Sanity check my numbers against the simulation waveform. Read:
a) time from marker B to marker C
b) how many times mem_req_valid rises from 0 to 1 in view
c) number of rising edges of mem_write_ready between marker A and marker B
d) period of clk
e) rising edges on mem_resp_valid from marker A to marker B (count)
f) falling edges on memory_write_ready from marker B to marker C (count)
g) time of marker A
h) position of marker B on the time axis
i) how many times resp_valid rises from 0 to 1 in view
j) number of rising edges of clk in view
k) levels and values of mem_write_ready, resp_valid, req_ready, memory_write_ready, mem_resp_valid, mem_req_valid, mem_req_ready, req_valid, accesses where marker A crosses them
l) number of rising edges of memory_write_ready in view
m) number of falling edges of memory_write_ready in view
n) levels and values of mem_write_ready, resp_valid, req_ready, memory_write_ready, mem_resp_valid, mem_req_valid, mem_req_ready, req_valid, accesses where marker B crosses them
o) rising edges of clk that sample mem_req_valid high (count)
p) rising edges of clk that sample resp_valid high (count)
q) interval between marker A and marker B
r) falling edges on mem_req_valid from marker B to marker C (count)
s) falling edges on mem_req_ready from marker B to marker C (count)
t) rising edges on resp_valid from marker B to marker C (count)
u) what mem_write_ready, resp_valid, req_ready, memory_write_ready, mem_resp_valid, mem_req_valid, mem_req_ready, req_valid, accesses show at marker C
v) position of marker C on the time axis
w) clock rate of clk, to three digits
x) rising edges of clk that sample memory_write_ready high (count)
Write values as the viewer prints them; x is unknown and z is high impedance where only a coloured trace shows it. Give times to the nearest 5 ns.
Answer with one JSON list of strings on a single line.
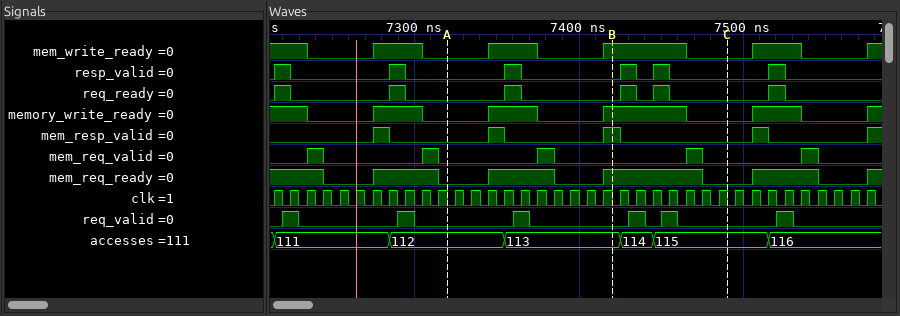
["70 ns", "5", "2", "10 ns", "2", "1", "7320 ns", "7420 ns", "6", "37", "mem_write_ready=0, resp_valid=0, req_ready=0, memory_write_ready=0, mem_resp_valid=0, mem_req_valid=0, mem_req_ready=0, req_valid=0, accesses=112", "5", "5", "mem_write_ready=1, resp_valid=0, req_ready=0, memory_write_ready=1, mem_resp_valid=1, mem_req_valid=0, mem_req_ready=1, req_valid=0, accesses=113", "5", "6", "100 ns", "1", "1", "2", "mem_write_ready=0, resp_valid=0, req_ready=0, memory_write_ready=0, mem_resp_valid=0, mem_req_valid=0, mem_req_ready=0, req_valid=0, accesses=115", "7490 ns", "100 MHz", "17"]
